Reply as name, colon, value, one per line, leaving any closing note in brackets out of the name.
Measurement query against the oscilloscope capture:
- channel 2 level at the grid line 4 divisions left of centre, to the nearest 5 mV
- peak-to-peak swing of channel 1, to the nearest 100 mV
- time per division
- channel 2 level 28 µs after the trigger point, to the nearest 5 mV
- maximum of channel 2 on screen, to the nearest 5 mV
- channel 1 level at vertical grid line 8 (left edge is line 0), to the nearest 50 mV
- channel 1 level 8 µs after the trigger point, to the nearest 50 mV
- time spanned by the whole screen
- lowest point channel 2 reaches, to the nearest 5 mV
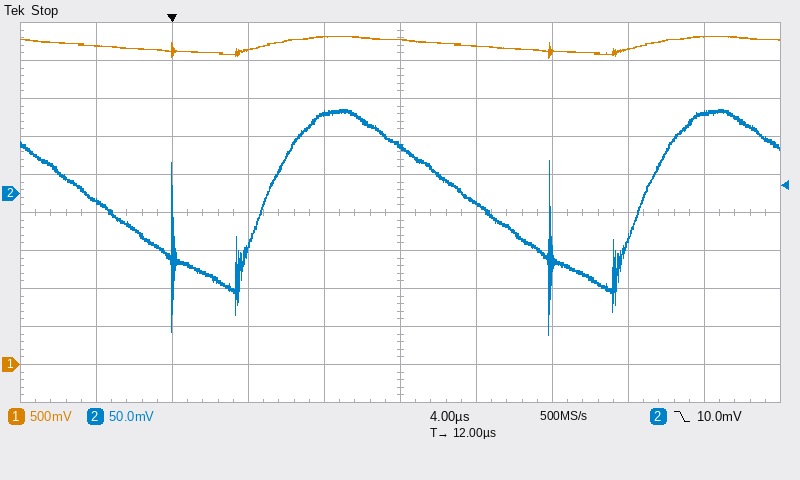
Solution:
channel 2 level at the grid line 4 divisions left of centre, to the nearest 5 mV: -10 mV
peak-to-peak swing of channel 1, to the nearest 100 mV: 300 mV
time per division: 4 µs
channel 2 level 28 µs after the trigger point, to the nearest 5 mV: 105 mV
maximum of channel 2 on screen, to the nearest 5 mV: 110 mV
channel 1 level at vertical grid line 8 (left edge is line 0), to the nearest 50 mV: 4.15 V
channel 1 level 8 µs after the trigger point, to the nearest 50 mV: 4.30 V
time spanned by the whole screen: 40 µs
lowest point channel 2 reaches, to the nearest 5 mV: -185 mV
